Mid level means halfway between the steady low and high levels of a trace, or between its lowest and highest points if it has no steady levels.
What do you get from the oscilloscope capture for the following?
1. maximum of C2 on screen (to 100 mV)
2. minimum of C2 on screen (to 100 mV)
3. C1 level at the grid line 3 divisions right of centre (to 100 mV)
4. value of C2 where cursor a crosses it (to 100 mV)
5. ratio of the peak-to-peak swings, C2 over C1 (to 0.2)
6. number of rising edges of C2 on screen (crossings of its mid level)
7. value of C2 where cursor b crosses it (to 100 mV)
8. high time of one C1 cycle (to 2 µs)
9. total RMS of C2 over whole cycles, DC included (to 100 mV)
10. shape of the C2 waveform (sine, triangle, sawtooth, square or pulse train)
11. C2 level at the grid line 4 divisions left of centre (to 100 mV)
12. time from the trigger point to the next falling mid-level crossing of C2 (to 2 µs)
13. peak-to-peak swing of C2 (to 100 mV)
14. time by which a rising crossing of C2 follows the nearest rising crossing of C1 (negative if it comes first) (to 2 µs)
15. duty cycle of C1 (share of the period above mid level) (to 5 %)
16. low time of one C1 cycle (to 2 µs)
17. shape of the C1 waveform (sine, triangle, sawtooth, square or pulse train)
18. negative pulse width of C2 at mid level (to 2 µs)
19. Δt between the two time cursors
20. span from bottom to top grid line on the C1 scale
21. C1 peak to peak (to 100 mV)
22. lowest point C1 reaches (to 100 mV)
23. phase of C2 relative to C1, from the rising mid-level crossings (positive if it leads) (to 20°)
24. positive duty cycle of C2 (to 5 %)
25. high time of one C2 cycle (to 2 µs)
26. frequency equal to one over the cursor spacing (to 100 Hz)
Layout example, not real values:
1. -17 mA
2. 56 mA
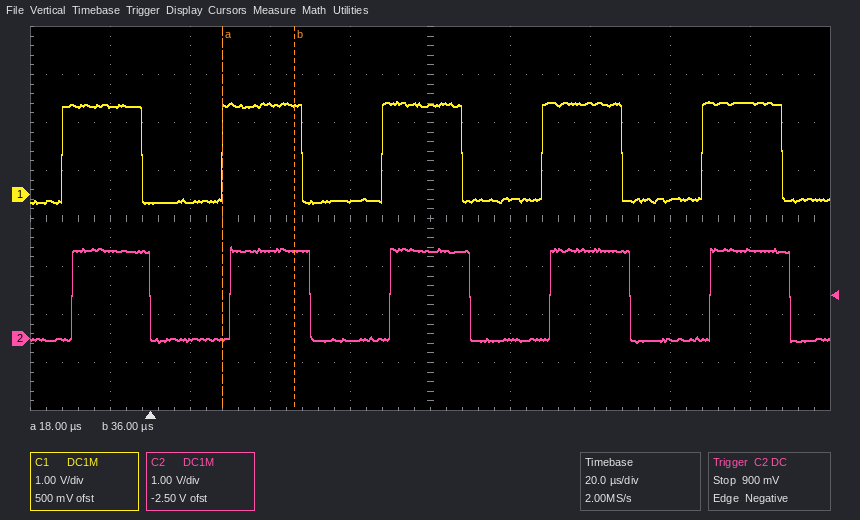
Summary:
1. 1.9 V
2. -100 mV
3. -100 mV
4. 0.0 V
5. 1.0
6. 5
7. 1.8 V
8. 20 µs
9. 1.3 V
10. square
11. 1.8 V
12. 40 µs
13. 2.0 V
14. +2 µs
15. 50 %
16. 20 µs
17. square
18. 20 µs
19. 18 µs
20. 8 V
21. 2.1 V
22. -200 mV
23. -20°
24. 50 %
25. 20 µs
26. 55.6 kHz
